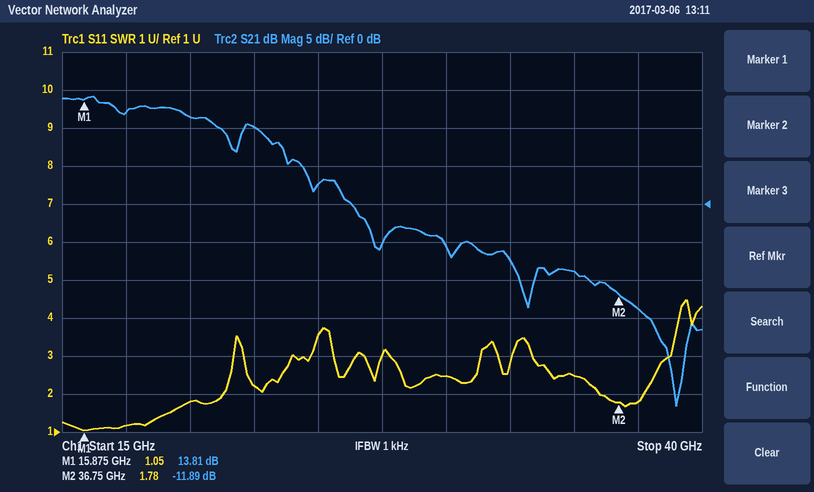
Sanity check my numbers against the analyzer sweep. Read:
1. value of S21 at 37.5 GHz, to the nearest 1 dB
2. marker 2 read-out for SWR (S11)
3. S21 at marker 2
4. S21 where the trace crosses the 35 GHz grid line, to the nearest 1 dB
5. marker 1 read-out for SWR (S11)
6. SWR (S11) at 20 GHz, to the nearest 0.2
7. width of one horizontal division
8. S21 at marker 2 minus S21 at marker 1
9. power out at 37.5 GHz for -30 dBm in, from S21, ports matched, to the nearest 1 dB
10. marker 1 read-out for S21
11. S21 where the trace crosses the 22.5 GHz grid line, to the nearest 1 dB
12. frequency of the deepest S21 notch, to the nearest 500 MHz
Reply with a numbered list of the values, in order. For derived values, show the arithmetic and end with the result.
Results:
1. -14 dB
2. 1.78
3. -11.89 dB
4. -9 dB
5. 1.05
6. 1.8
7. 2.5 GHz
8. -11.89 − (13.81) = -25.70 dB
9. -30 dBm + (-14 dB) = -44 dBm
10. 13.81 dB
11. 10 dB
12. 39.0 GHz
